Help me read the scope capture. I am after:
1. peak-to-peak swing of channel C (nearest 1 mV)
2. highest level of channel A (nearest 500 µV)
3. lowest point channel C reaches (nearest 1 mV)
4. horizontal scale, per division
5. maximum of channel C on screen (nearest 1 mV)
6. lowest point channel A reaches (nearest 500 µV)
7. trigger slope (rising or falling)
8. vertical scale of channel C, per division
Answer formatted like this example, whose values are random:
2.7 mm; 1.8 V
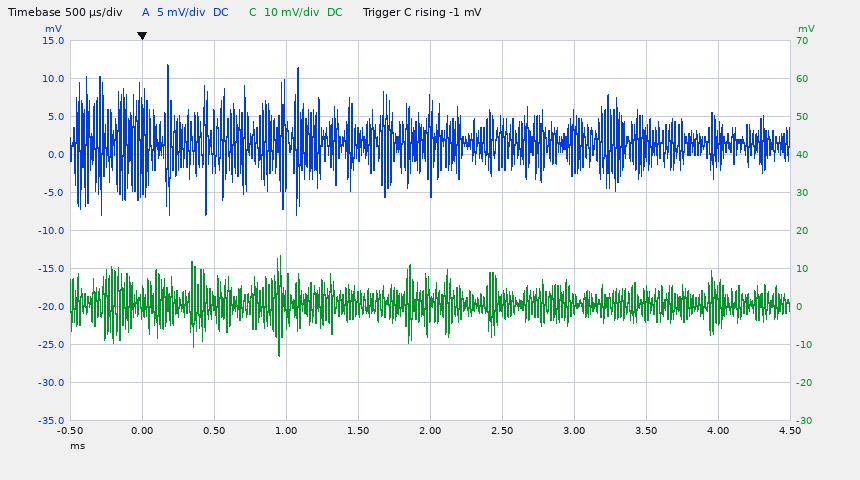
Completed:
26 mV; 12.0 mV; -13 mV; 500 µs; 13 mV; -8.0 mV; rising; 10 mV
